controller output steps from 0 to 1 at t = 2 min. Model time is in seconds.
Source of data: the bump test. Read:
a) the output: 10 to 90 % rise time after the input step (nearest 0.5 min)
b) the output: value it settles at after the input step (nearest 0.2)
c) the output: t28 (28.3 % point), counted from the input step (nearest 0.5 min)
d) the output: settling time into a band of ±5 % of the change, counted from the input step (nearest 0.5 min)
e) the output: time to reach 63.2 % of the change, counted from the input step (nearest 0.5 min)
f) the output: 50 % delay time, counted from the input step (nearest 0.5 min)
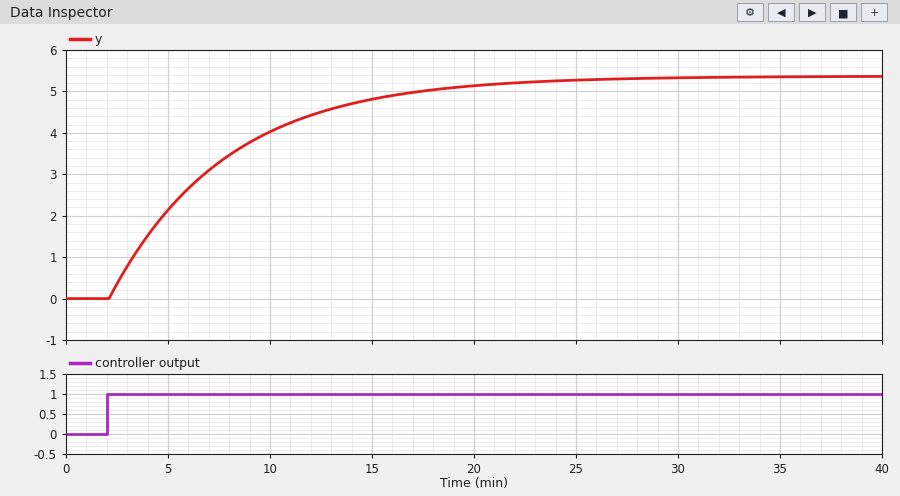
12.5 min
5.4
2.0 min
17.0 min
6.0 min
4.0 min
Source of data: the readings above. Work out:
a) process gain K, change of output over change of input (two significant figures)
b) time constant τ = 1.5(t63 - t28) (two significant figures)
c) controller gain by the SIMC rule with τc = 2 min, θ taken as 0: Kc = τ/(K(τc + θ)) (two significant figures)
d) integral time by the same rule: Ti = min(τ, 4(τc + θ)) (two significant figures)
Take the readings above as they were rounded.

5.4
6.0 min
0.56
6.0 min
